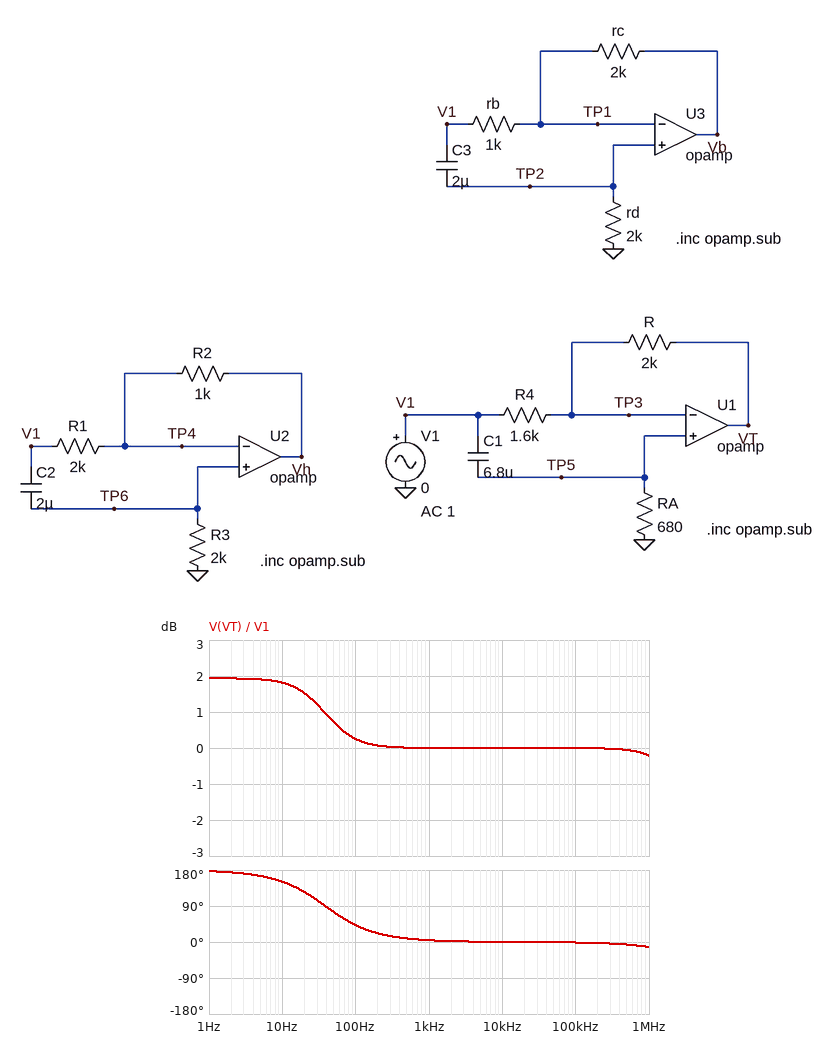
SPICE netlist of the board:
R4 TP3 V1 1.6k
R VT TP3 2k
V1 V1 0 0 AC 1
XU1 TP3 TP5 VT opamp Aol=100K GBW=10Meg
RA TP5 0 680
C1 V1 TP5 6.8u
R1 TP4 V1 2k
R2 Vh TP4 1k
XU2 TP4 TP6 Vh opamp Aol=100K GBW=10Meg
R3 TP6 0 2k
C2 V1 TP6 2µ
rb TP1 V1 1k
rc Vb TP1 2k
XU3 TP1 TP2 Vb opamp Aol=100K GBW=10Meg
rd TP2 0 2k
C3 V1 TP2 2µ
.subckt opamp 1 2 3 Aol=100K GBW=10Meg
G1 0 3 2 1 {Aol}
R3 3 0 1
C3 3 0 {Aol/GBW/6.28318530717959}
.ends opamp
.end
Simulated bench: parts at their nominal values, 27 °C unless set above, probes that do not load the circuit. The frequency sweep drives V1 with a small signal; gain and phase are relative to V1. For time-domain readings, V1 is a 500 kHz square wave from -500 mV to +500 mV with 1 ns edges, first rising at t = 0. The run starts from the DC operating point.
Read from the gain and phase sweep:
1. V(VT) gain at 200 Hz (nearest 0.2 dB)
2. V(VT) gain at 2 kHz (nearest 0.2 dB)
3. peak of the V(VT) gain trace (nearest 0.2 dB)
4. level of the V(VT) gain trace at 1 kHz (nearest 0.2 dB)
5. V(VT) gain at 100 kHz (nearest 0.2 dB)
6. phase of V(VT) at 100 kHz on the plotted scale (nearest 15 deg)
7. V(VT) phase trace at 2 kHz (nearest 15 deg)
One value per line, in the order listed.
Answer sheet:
0 dB
0 dB
2.0 dB
0 dB
0 dB
0 deg
0 deg
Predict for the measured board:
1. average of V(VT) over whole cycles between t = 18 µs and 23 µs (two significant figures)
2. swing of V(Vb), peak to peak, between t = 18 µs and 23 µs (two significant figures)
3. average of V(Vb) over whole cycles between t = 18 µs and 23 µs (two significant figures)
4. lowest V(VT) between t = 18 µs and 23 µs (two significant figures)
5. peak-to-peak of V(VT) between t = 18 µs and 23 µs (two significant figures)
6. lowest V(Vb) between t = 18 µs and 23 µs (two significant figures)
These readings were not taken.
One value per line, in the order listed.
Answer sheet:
1.1 V
1.0 V
1.5 V
620 mV
1.0 V
990 mV
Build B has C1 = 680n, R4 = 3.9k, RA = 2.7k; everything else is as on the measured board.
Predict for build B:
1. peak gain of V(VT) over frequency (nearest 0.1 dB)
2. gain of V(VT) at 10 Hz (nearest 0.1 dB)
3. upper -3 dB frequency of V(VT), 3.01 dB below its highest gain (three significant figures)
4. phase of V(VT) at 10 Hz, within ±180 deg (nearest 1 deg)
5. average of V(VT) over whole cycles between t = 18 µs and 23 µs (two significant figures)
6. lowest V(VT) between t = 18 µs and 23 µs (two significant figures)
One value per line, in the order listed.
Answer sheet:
0 dB
-5.6 dB
6.61 MHz
161 deg
750 mV
250 mV
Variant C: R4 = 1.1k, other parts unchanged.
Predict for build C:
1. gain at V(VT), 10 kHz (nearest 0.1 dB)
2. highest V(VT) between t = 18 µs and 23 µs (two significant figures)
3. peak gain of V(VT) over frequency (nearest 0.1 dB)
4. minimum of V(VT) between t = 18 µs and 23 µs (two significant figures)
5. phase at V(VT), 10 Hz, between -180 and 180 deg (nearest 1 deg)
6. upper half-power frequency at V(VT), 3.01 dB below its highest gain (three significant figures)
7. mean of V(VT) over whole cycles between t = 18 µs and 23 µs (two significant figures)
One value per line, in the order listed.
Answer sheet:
0 dB
1.9 V
5.2 dB
900 mV
155 deg
54.8 Hz
1.4 V
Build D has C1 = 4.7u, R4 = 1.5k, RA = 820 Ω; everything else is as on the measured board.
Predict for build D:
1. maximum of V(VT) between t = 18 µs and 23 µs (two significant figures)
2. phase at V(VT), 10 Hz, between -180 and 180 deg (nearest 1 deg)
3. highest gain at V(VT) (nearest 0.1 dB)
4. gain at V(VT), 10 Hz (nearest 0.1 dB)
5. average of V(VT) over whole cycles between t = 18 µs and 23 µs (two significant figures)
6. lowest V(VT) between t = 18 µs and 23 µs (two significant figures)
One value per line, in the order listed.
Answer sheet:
1.7 V
156 deg
2.5 dB
2.4 dB
1.2 V
660 mV
